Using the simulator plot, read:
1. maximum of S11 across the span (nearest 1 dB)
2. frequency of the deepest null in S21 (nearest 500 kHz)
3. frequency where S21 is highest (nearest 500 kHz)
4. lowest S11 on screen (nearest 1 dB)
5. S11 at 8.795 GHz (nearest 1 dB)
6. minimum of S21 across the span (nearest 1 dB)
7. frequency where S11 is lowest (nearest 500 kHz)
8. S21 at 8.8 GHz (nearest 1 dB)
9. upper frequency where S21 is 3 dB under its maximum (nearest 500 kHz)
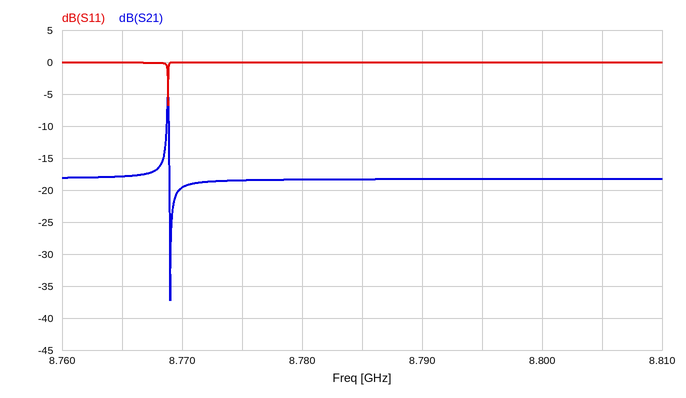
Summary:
0 dB
8.7690 GHz
8.7690 GHz
-7 dB
0 dB
-37 dB
8.7690 GHz
-18 dB
8.7690 GHz
